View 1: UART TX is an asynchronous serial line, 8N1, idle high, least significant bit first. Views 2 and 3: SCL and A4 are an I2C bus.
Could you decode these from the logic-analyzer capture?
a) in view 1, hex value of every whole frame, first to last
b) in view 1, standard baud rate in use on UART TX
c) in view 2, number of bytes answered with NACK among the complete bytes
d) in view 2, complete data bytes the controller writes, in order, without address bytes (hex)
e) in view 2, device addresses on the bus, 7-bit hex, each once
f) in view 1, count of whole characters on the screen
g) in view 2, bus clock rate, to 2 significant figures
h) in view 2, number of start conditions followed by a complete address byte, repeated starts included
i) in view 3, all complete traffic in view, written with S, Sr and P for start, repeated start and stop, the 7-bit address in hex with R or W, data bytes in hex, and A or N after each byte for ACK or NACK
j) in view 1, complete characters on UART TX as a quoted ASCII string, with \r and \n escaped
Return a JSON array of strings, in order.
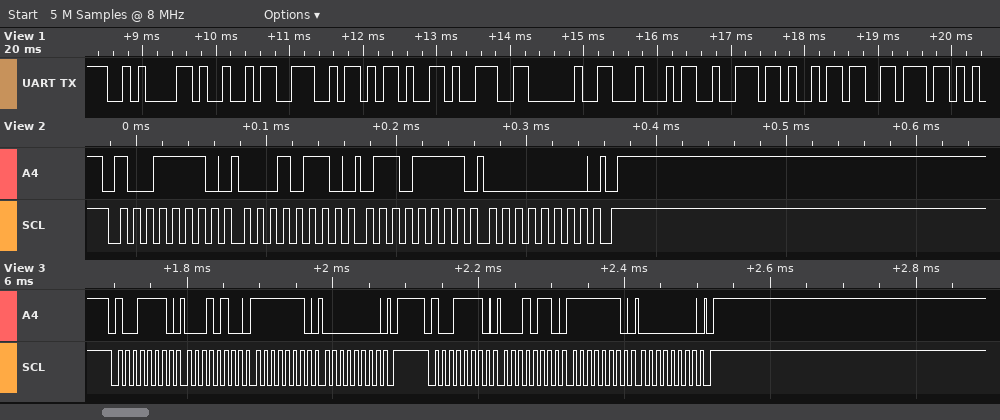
["0x0A 0x49 0x4E 0x2D 0x39 0x20 0x44 0x72 0x69 0x76", "9600 baud", "0", "16 6F 00", "0x4F", "10", "100 kHz", "1", "S 4FW A 14 A FE A 00 A P S 4FW A 16 A FE A 00 A P", "\"\\nIN-9 Driv\""]
